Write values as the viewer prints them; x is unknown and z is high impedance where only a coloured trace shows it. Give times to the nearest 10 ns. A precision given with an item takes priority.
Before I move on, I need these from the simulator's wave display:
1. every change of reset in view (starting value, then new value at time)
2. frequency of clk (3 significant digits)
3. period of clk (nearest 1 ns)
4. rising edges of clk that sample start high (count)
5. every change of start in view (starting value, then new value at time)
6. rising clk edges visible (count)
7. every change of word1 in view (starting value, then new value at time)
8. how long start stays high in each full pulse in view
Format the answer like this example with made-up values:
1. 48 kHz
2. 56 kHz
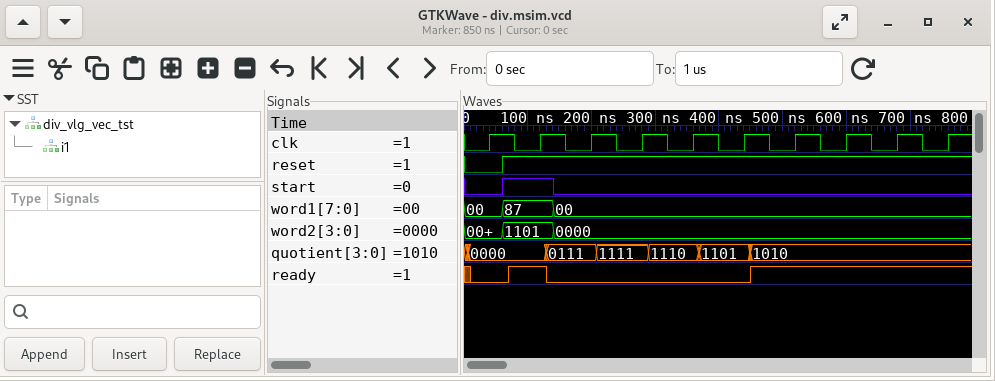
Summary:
1. 0, 1 at 60 ns
2. 12.5 MHz
3. 80 ns
4. 1
5. 0, 1 at 60 ns, 0 at 140 ns
6. 10
7. 00, 87 at 60 ns, 00 at 140 ns
8. 80 ns
